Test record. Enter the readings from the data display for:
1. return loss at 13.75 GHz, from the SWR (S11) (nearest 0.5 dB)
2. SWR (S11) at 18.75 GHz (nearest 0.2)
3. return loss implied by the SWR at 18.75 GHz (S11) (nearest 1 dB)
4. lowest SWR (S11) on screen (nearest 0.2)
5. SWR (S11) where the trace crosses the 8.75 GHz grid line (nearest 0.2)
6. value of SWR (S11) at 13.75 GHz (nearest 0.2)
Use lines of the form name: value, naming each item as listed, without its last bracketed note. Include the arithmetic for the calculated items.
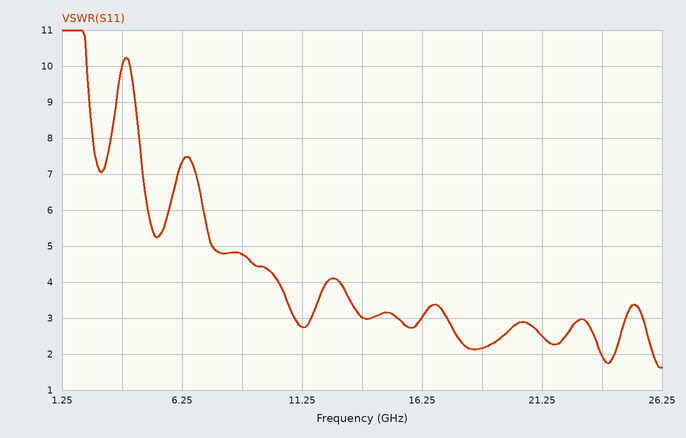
return loss at 13.75 GHz, from the SWR (S11): −20 log10((3 − 1)/(3 + 1)) ≈ 6.0 dB
SWR (S11) at 18.75 GHz: 2.2
return loss implied by the SWR at 18.75 GHz (S11): −20 log10((2.2 − 1)/(2.2 + 1)) ≈ 9 dB
lowest SWR (S11) on screen: 1.6
SWR (S11) where the trace crosses the 8.75 GHz grid line: 4.8
value of SWR (S11) at 13.75 GHz: 3.0
